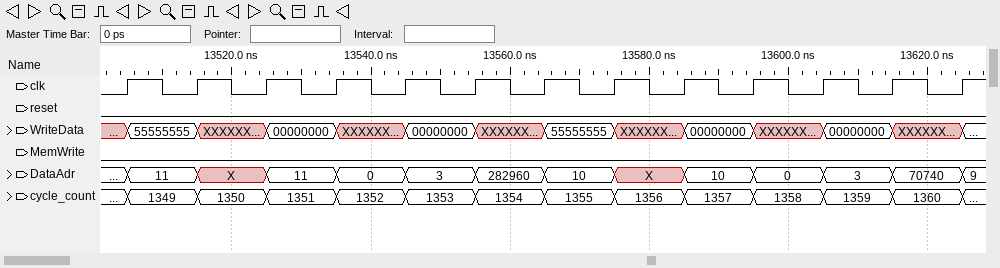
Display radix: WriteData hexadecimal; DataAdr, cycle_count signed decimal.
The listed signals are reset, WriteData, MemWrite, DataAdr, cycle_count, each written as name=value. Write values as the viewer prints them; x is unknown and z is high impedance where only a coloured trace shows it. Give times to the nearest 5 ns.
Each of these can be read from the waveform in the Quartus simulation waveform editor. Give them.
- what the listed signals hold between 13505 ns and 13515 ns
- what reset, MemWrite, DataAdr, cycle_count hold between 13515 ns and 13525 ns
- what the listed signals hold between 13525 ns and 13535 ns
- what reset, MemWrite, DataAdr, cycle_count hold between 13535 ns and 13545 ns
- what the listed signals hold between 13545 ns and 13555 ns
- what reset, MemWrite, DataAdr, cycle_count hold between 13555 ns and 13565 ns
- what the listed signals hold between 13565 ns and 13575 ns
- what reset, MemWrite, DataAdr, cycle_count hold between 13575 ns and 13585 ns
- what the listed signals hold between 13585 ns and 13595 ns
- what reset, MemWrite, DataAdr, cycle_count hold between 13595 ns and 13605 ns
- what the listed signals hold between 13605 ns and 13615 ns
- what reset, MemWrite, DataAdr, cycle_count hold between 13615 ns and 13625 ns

reset=0, WriteData=55555555, MemWrite=0, DataAdr=11, cycle_count=1349
reset=0, MemWrite=0, DataAdr=X, cycle_count=1350
reset=0, WriteData=00000000, MemWrite=0, DataAdr=11, cycle_count=1351
reset=0, MemWrite=0, DataAdr=0, cycle_count=1352
reset=0, WriteData=00000000, MemWrite=0, DataAdr=3, cycle_count=1353
reset=0, MemWrite=0, DataAdr=282960, cycle_count=1354
reset=0, WriteData=55555555, MemWrite=0, DataAdr=10, cycle_count=1355
reset=0, MemWrite=0, DataAdr=X, cycle_count=1356
reset=0, WriteData=00000000, MemWrite=0, DataAdr=10, cycle_count=1357
reset=0, MemWrite=0, DataAdr=0, cycle_count=1358
reset=0, WriteData=00000000, MemWrite=0, DataAdr=3, cycle_count=1359
reset=0, MemWrite=0, DataAdr=70740, cycle_count=1360
